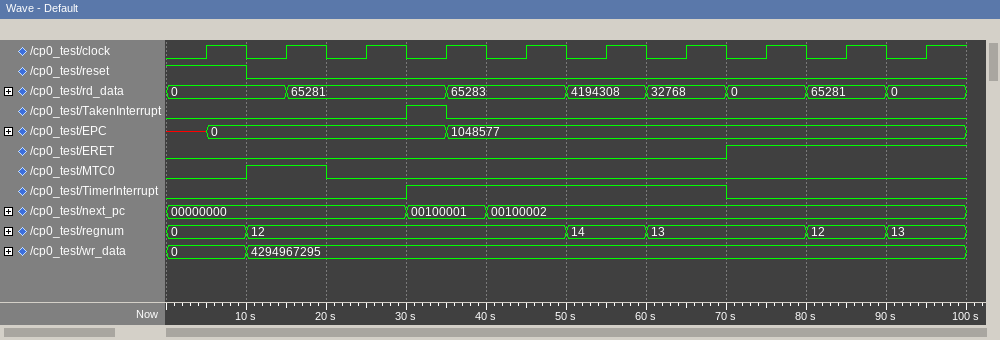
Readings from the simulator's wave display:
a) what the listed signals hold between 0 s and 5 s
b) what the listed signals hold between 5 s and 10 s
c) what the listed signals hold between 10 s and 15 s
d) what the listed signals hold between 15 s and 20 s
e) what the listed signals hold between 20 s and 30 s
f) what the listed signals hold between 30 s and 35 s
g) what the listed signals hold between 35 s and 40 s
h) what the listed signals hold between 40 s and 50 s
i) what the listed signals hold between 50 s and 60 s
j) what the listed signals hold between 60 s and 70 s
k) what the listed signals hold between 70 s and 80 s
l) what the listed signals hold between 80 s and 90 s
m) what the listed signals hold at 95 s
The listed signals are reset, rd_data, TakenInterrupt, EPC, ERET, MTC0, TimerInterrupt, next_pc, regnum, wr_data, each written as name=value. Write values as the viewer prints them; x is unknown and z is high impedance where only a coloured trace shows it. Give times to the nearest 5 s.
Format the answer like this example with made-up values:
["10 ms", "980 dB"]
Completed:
["reset=1, rd_data=0, TakenInterrupt=0, EPC=x, ERET=0, MTC0=0, TimerInterrupt=0, next_pc=00000000, regnum=0, wr_data=0", "reset=1, rd_data=0, TakenInterrupt=0, EPC=0, ERET=0, MTC0=0, TimerInterrupt=0, next_pc=00000000, regnum=0, wr_data=0", "reset=0, rd_data=0, TakenInterrupt=0, EPC=0, ERET=0, MTC0=1, TimerInterrupt=0, next_pc=00000000, regnum=12, wr_data=4294967295", "reset=0, rd_data=65281, TakenInterrupt=0, EPC=0, ERET=0, MTC0=1, TimerInterrupt=0, next_pc=00000000, regnum=12, wr_data=4294967295", "reset=0, rd_data=65281, TakenInterrupt=0, EPC=0, ERET=0, MTC0=0, TimerInterrupt=0, next_pc=00000000, regnum=12, wr_data=4294967295", "reset=0, rd_data=65281, TakenInterrupt=1, EPC=0, ERET=0, MTC0=0, TimerInterrupt=1, next_pc=00100001, regnum=12, wr_data=4294967295", "reset=0, rd_data=65283, TakenInterrupt=0, EPC=1048577, ERET=0, MTC0=0, TimerInterrupt=1, next_pc=00100001, regnum=12, wr_data=4294967295", "reset=0, rd_data=65283, TakenInterrupt=0, EPC=1048577, ERET=0, MTC0=0, TimerInterrupt=1, next_pc=00100002, regnum=12, wr_data=4294967295", "reset=0, rd_data=4194308, TakenInterrupt=0, EPC=1048577, ERET=0, MTC0=0, TimerInterrupt=1, next_pc=00100002, regnum=14, wr_data=4294967295", "reset=0, rd_data=32768, TakenInterrupt=0, EPC=1048577, ERET=0, MTC0=0, TimerInterrupt=1, next_pc=00100002, regnum=13, wr_data=4294967295", "reset=0, rd_data=0, TakenInterrupt=0, EPC=1048577, ERET=1, MTC0=0, TimerInterrupt=0, next_pc=00100002, regnum=13, wr_data=4294967295", "reset=0, rd_data=65281, TakenInterrupt=0, EPC=1048577, ERET=1, MTC0=0, TimerInterrupt=0, next_pc=00100002, regnum=12, wr_data=4294967295", "reset=0, rd_data=0, TakenInterrupt=0, EPC=1048577, ERET=1, MTC0=0, TimerInterrupt=0, next_pc=00100002, regnum=13, wr_data=4294967295"]
